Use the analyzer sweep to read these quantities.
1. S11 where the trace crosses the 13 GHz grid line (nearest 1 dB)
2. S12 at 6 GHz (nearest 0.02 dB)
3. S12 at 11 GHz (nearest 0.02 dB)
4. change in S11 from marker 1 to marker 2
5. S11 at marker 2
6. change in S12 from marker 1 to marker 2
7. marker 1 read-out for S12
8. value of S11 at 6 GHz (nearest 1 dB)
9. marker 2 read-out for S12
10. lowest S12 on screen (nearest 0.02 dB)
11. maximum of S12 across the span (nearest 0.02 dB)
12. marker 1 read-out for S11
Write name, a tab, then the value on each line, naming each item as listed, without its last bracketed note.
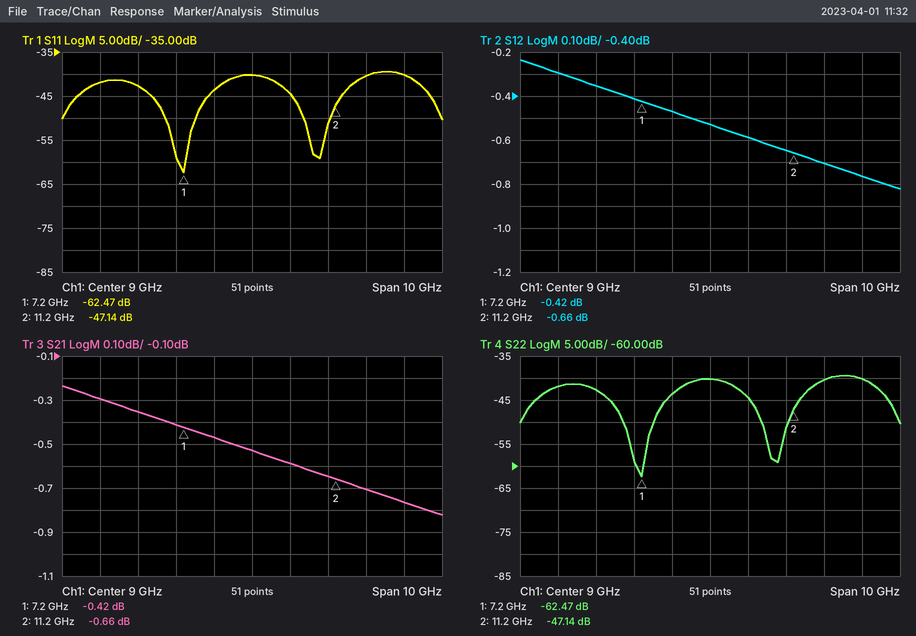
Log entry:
S11 where the trace crosses the 13 GHz grid line	-40 dB
S12 at 6 GHz	-0.36 dB
S12 at 11 GHz	-0.64 dB
change in S11 from marker 1 to marker 2	15.33 dB
S11 at marker 2	-47.14 dB
change in S12 from marker 1 to marker 2	-0.24 dB
marker 1 read-out for S12	-0.42 dB
value of S11 at 6 GHz	-43 dB
marker 2 read-out for S12	-0.66 dB
lowest S12 on screen	-0.82 dB
maximum of S12 across the span	-0.24 dB
marker 1 read-out for S11	-62.47 dB
